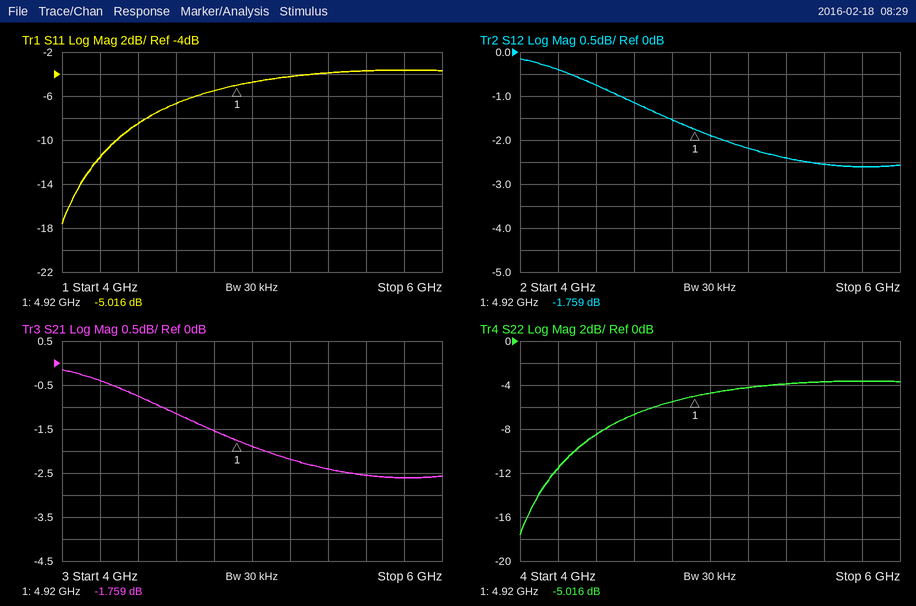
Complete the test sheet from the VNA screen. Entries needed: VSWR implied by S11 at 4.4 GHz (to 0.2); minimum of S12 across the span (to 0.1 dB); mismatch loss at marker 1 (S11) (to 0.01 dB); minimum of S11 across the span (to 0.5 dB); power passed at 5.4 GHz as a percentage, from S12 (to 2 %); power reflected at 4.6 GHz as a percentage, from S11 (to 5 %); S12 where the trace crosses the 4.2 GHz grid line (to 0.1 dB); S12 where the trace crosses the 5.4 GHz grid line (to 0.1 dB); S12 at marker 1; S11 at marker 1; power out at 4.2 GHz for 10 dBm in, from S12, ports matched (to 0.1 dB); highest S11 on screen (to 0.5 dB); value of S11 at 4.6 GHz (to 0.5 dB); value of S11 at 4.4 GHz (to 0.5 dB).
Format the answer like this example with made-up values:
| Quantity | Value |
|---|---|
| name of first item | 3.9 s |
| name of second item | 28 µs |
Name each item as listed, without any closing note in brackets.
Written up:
| Quantity | Value |
|---|---|
| VSWR implied by S11 at 4.4 GHz | 2.2 |
| minimum of S12 across the span | -2.6 dB |
| mismatch loss at marker 1 (S11) | 1.64 dB |
| minimum of S11 across the span | -17.5 dB |
| power passed at 5.4 GHz as a percentage, from S12 | 58 % |
| power reflected at 4.6 GHz as a percentage, from S11 | 20 % |
| S12 where the trace crosses the 4.2 GHz grid line | -0.4 dB |
| S12 where the trace crosses the 5.4 GHz grid line | -2.4 dB |
| S12 at marker 1 | -1.759 dB |
| S11 at marker 1 | -5.016 dB |
| power out at 4.2 GHz for 10 dBm in, from S12, ports matched | 9.6 dBm |
| highest S11 on screen | -3.5 dB |
| value of S11 at 4.6 GHz | -6.5 dB |
| value of S11 at 4.4 GHz | -8.5 dB |
